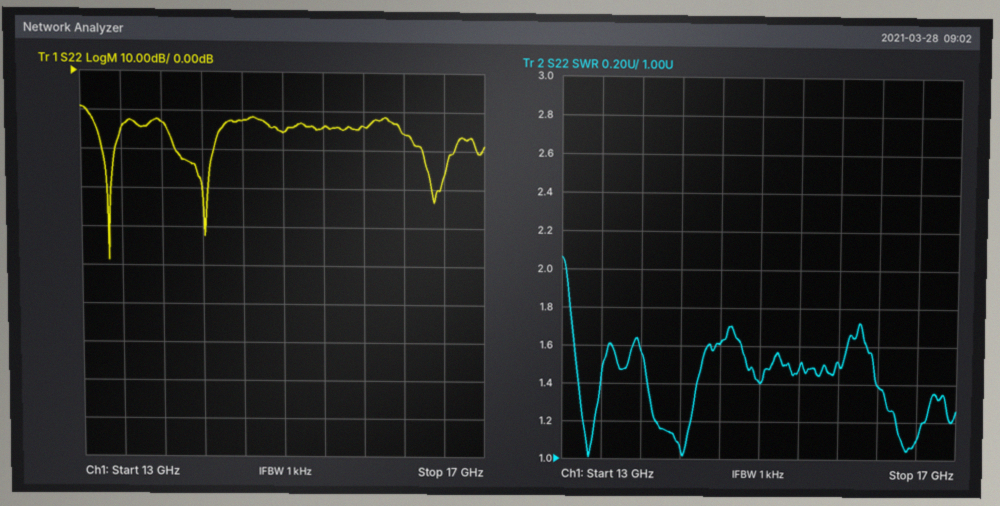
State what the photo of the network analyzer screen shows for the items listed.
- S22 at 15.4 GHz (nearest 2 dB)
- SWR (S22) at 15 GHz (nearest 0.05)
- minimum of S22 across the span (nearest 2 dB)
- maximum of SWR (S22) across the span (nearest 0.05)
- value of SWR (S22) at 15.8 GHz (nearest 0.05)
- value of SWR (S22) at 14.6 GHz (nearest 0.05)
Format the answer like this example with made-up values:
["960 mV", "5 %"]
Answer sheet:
["-14 dB", "1.40", "-48 dB", "2.05", "1.50", "1.60"]
